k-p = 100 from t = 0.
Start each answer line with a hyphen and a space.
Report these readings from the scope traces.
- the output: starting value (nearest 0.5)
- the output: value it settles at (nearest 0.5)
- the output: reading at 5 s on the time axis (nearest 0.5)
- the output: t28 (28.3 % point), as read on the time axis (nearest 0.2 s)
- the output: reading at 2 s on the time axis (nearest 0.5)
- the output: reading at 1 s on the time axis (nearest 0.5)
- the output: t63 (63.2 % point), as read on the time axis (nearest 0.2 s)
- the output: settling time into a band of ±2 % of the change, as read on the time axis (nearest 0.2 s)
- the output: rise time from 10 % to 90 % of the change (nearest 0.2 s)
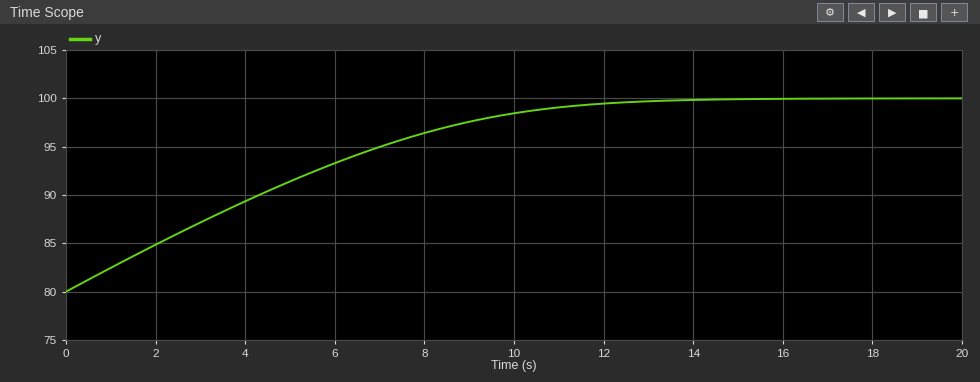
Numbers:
- 80.0
- 100.0
- 91.5
- 2.4 s
- 85.0
- 82.5
- 5.6 s
- 12.6 s
- 8.6 s
